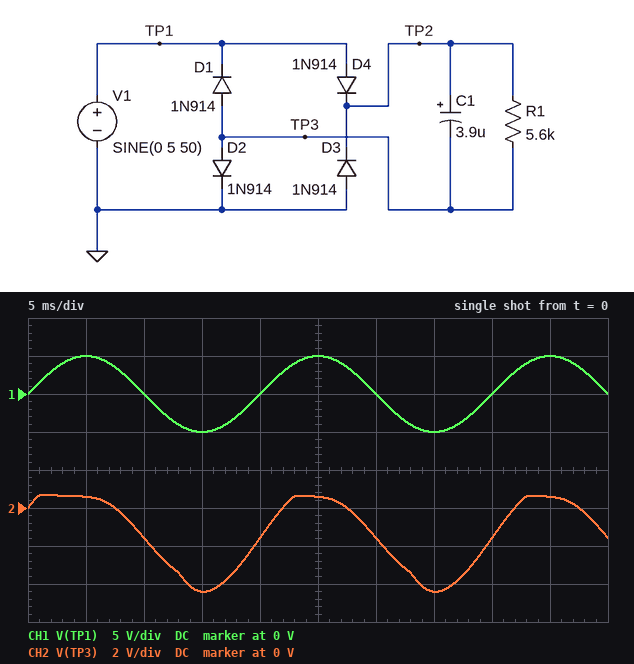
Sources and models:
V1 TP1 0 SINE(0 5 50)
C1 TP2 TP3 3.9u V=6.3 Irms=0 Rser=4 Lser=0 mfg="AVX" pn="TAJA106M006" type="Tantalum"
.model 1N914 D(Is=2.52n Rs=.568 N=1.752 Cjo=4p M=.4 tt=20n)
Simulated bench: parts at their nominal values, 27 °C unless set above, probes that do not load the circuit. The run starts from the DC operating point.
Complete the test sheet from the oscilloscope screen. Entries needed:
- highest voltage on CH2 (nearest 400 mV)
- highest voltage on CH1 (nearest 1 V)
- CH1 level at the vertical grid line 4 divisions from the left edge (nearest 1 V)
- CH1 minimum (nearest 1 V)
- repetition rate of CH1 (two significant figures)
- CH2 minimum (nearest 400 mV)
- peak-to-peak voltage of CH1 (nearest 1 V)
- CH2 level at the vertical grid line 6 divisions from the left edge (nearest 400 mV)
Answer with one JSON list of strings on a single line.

["800 mV", "5 V", "0 V", "-5 V", "50 Hz", "-4.4 V", "10 V", "-1.6 V"]
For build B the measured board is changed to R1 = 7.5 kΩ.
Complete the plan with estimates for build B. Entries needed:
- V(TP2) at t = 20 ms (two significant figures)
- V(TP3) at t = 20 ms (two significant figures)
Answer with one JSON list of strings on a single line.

["1.7 V", "-1.7 V"]
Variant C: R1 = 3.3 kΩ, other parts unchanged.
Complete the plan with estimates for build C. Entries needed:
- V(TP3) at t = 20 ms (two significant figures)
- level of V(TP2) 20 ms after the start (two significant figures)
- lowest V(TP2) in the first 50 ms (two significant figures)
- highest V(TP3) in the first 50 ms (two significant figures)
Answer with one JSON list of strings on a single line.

["-1.4 V", "1.4 V", "-660 mV", "670 mV"]
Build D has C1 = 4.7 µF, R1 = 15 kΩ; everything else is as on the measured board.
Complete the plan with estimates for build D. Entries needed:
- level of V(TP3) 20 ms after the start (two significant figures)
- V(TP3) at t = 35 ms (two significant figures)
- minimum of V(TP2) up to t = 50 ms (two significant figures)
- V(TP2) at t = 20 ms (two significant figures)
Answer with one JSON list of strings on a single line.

["-1.8 V", "-4.4 V", "-620 mV", "1.8 V"]
